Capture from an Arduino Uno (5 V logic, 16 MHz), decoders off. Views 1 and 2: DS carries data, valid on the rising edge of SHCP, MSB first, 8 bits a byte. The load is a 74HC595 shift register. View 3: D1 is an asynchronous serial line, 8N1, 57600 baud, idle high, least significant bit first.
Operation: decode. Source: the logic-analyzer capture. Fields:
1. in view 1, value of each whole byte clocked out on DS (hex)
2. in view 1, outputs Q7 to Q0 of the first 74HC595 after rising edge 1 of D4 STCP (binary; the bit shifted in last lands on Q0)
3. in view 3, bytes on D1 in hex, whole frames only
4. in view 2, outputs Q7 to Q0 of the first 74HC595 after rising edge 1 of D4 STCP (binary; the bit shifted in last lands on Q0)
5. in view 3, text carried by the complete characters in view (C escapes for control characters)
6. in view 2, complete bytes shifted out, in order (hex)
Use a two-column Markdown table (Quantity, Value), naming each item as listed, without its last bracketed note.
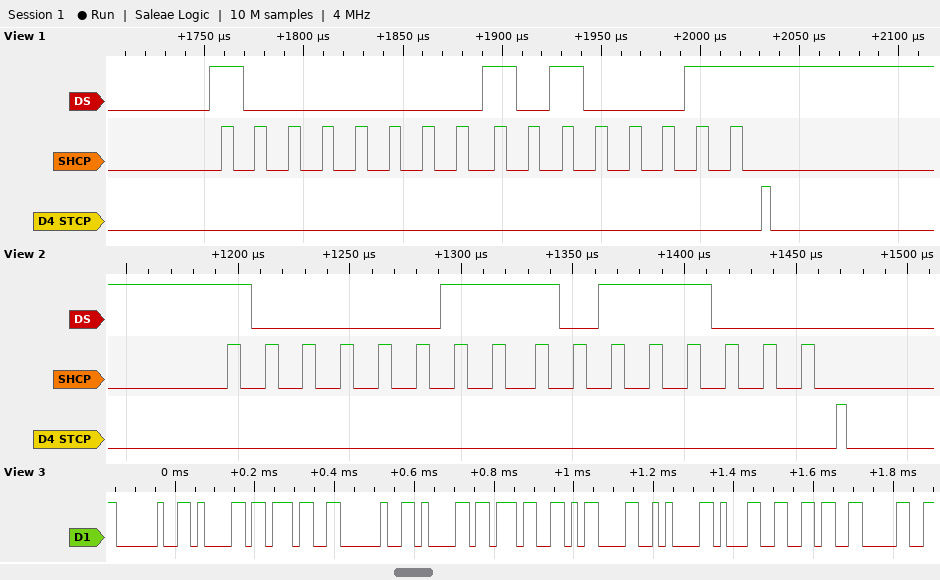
| Quantity | Value |
|---|---|
| in view 1, value of each whole byte clocked out on DS | 80 A3 |
| in view 1, outputs Q7 to Q0 of the first 74HC595 after rising edge 1 of D4 STCP | 10100011 |
| in view 3, bytes on D1 in hex, whole frames only | 20 61 37 20 61 37 0D 0A 31 36 30 |
| in view 2, outputs Q7 to Q0 of the first 74HC595 after rising edge 1 of D4 STCP | 10111000 |
| in view 3, text carried by the complete characters in view | " a7 a7\r\n160" |
| in view 2, complete bytes shifted out, in order | 83 B8 |
